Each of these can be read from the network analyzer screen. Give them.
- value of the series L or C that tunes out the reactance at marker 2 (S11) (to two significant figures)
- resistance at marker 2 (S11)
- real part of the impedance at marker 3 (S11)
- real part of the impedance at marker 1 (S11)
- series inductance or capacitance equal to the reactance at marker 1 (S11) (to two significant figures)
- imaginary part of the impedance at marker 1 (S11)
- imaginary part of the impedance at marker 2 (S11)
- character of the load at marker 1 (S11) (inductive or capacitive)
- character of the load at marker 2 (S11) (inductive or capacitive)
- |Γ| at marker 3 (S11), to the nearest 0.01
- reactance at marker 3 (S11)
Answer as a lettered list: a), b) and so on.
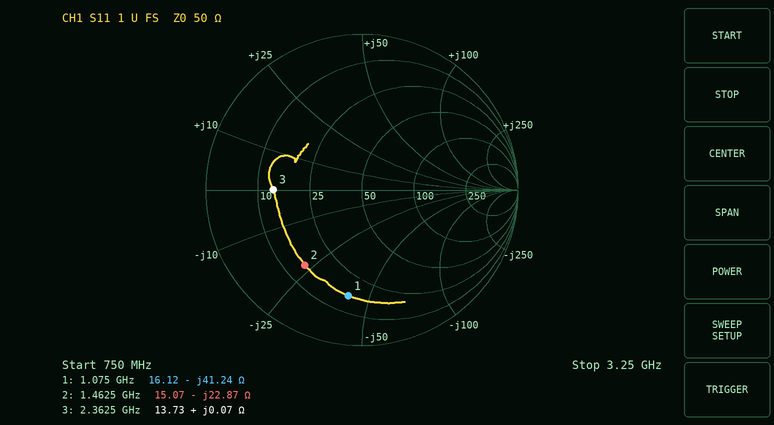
a) 2.5 nH
b) 15.07 Ω
c) 13.73 Ω
d) 16.12 Ω
e) 3.6 pF
f) -41.24 Ω
g) -22.87 Ω
h) capacitive
i) capacitive
j) 0.57
k) +0.07 Ω
